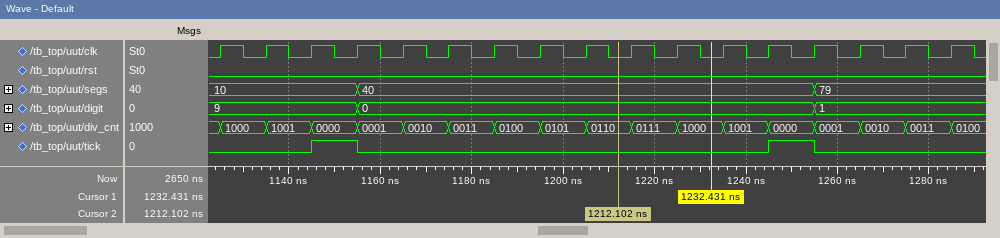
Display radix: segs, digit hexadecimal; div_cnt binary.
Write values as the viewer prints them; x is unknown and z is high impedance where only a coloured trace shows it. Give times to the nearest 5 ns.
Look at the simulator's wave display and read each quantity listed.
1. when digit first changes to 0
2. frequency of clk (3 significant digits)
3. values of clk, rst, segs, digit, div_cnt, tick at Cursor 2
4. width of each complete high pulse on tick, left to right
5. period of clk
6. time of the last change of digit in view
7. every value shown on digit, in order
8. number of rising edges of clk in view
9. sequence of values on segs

1155 ns
100 MHz
clk=0, rst=0, segs=40, digit=0, div_cnt=0110, tick=0
10 ns, 10 ns
10 ns
1255 ns
9, 0, 1
17
10, 40, 79
